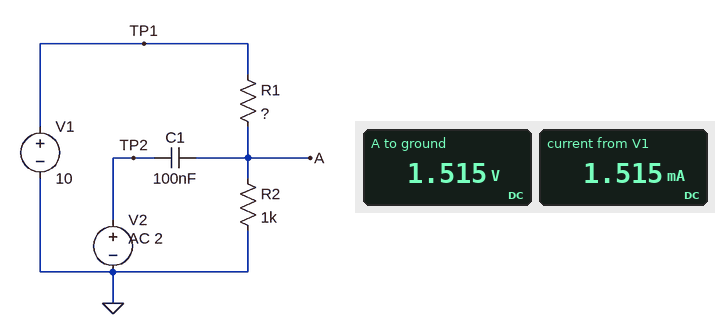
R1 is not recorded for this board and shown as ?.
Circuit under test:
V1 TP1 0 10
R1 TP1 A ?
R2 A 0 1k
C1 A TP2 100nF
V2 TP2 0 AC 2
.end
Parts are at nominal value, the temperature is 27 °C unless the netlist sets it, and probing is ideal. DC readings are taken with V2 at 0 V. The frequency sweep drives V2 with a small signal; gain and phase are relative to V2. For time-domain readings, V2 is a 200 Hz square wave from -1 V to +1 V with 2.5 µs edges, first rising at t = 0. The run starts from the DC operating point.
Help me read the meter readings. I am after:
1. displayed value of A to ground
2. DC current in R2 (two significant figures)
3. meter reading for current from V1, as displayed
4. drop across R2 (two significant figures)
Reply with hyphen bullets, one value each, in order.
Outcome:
- 1.515 V
- 1.5 mA
- 1.515 mA
- 1.5 V
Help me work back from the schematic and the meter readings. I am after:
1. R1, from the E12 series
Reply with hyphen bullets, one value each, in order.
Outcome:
- 5.6 kΩ
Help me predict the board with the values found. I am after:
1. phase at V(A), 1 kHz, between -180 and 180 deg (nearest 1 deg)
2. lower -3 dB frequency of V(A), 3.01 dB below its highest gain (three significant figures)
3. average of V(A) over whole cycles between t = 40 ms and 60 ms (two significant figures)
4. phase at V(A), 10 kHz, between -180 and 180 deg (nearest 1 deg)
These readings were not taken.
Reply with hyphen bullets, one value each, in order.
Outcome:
- 62 deg
- 1.88 kHz
- 1.5 V
- 11 deg
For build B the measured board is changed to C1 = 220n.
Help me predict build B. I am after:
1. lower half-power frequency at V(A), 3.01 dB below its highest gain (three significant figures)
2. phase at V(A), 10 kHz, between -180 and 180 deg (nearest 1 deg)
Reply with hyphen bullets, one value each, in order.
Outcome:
- 853 Hz
- 5 deg
